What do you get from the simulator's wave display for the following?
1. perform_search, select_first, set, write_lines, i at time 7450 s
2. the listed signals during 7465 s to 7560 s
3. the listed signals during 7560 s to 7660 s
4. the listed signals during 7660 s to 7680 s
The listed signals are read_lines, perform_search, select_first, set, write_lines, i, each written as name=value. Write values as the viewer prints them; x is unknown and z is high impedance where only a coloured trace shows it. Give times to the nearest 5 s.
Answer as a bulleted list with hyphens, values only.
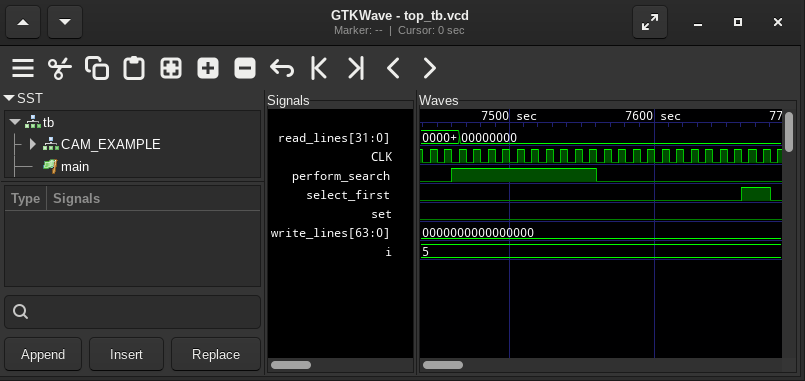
- perform_search=0, select_first=0, set=0, write_lines=0000000000000000, i=5
- read_lines=00000000, perform_search=1, select_first=0, set=0, write_lines=0000000000000000, i=5
- read_lines=00000000, perform_search=0, select_first=0, set=0, write_lines=0000000000000000, i=5
- read_lines=00000000, perform_search=0, select_first=1, set=0, write_lines=0000000000000000, i=5
